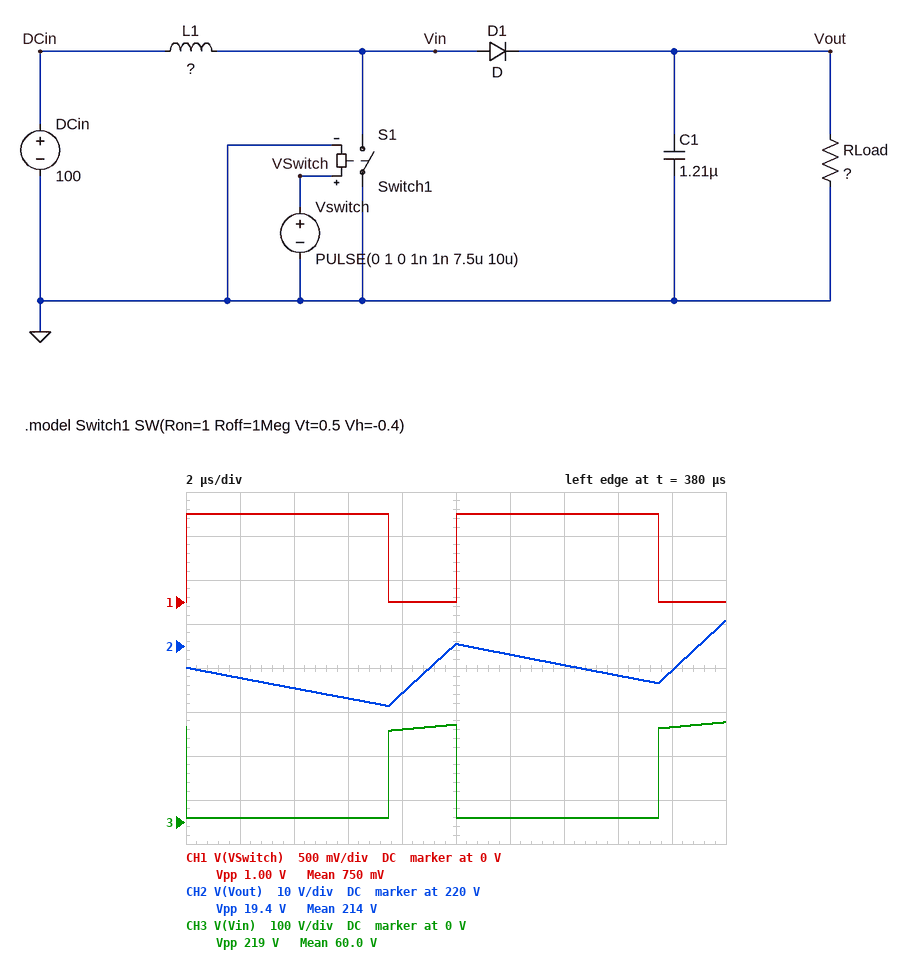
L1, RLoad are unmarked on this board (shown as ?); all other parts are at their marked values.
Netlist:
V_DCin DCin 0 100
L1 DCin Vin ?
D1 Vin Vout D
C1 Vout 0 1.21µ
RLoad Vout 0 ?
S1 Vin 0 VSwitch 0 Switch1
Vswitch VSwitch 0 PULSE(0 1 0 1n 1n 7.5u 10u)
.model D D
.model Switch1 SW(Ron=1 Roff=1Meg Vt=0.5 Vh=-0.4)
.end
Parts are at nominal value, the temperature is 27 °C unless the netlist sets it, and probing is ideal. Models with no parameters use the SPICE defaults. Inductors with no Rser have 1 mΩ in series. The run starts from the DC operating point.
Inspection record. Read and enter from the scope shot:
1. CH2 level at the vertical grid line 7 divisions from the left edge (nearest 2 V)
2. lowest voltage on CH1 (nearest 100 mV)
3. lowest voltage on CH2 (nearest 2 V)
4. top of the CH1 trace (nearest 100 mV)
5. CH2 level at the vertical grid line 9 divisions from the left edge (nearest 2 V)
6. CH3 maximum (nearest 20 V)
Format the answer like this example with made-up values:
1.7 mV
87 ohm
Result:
216 V
0 V
206 V
1.0 V
214 V
220 V
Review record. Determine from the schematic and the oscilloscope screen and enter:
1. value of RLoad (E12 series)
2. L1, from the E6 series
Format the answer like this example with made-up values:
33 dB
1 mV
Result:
150 Ω
3.3 mH
